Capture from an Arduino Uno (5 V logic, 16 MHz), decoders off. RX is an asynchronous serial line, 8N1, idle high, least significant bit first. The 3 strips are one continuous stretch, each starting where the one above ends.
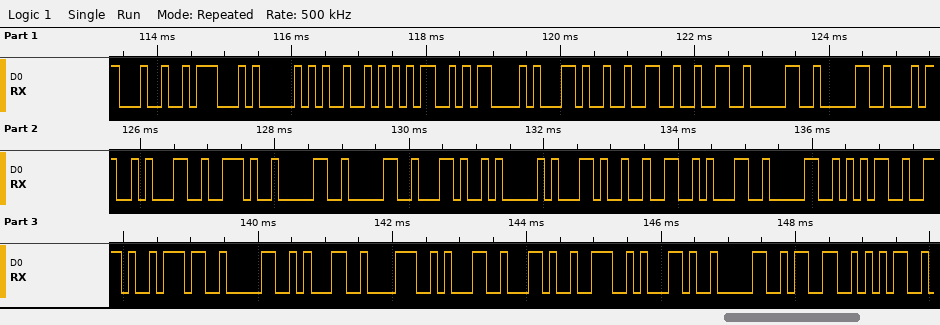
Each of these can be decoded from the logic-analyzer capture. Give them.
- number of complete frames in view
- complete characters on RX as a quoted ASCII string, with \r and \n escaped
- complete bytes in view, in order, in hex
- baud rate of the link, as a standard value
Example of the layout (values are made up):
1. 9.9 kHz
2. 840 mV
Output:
1. 35
2. "$GPRMC,220041.00,A,2105.70181,N,035"
3. 0x24 0x47 0x50 0x52 0x4D 0x43 0x2C 0x32 0x32 0x30 0x30 0x34 0x31 0x2E 0x30 0x30 0x2C 0x41 0x2C 0x32 0x31 0x30 0x35 0x2E 0x37 0x30 0x31 0x38 0x31 0x2C 0x4E 0x2C 0x30 0x33 0x35
4. 9600 baud
